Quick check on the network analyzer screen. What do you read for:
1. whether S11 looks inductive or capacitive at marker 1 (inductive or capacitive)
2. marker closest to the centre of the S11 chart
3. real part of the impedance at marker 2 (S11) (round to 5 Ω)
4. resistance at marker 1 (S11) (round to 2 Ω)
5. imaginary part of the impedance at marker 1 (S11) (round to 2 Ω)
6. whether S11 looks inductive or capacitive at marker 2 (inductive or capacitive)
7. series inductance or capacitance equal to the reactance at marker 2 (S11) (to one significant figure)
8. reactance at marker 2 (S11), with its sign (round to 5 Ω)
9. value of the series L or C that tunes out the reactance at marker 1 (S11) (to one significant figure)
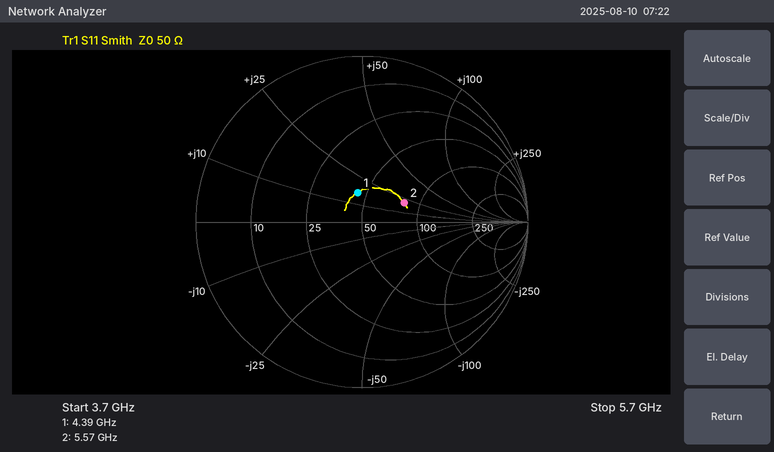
inductive
marker 1
80 Ω
44 Ω
+16 Ω
inductive
600 pH
+20 Ω
2 pF
